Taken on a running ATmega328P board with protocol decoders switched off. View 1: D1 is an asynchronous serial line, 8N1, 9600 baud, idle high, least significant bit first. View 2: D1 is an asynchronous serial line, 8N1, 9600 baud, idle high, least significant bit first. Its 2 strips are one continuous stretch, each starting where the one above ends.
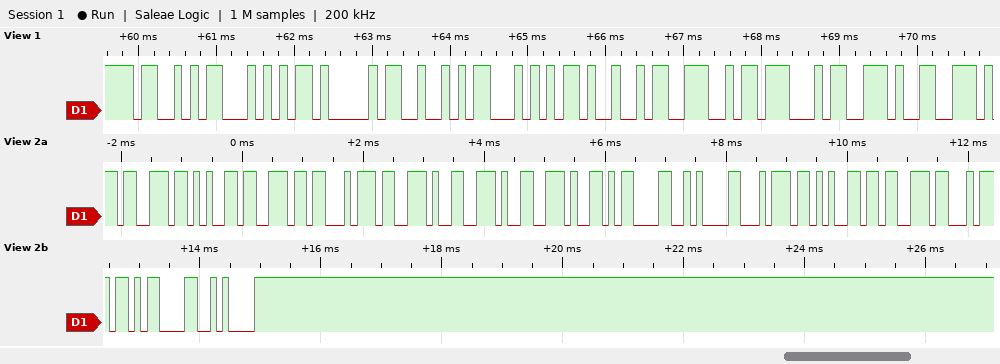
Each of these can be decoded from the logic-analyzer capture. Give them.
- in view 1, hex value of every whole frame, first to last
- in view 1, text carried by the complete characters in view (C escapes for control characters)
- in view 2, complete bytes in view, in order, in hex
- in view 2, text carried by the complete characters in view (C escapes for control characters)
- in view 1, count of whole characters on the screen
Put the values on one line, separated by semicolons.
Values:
53 54 41 52 54 49 4E 47 2E; "STARTING."; 73 65 6E 74 2E 2E 2E 0D 0A 74 65 73 74 0D 0A; "sent...\r\ntest\r\n"; 9
